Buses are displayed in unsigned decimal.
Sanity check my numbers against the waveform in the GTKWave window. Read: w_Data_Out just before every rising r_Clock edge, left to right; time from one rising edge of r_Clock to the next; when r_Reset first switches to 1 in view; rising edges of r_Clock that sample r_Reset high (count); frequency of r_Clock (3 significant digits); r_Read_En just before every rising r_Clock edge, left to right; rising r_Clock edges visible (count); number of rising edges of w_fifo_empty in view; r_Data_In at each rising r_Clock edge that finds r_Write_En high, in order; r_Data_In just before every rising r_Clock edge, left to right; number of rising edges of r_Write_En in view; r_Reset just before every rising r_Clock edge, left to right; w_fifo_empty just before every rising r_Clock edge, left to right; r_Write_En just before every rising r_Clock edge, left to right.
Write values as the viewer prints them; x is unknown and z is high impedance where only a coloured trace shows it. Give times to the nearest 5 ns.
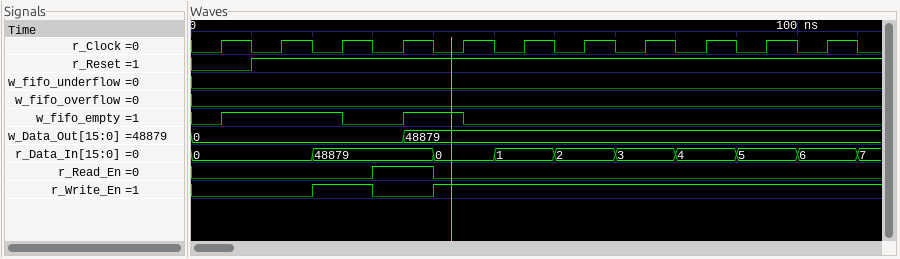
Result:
0, 0, 0, 0, 48879, 48879, 48879, 48879, 48879, 48879, 48879
10 ns
10 ns
10
100 MHz
0 0 0 1 0 0 0 0 0 0 0
11
2
48879, 0, 1, 2, 3, 4, 5, 6
0, 0, 48879, 48879, 0, 1, 2, 3, 4, 5, 6
2
0 1 1 1 1 1 1 1 1 1 1
0 1 1 0 1 0 0 0 0 0 0
0 0 1 0 1 1 1 1 1 1 1
